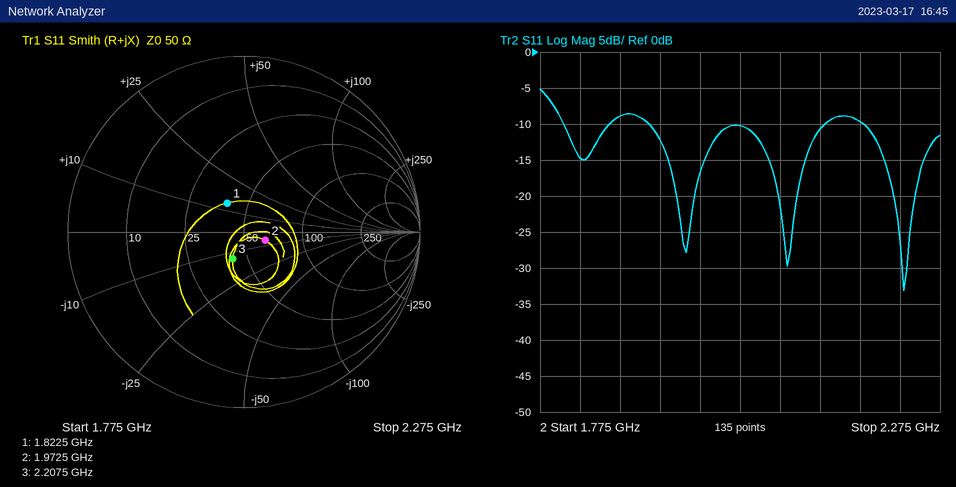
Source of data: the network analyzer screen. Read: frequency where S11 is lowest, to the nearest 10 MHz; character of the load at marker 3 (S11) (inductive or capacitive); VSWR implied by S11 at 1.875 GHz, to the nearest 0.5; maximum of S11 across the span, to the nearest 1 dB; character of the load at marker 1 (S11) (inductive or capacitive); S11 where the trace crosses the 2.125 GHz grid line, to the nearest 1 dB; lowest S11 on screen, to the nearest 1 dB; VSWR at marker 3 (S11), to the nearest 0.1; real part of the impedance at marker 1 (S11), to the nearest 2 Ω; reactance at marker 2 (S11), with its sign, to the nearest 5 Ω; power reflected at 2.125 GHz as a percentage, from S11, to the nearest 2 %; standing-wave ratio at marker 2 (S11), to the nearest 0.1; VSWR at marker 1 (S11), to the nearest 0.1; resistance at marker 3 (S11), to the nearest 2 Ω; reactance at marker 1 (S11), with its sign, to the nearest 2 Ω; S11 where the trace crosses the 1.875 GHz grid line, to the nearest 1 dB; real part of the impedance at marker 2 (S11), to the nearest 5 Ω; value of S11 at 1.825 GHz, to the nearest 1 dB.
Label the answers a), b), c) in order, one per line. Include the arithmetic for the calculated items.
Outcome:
a) 2.23 GHz
b) capacitive
c) |Γ| = 10^(-9/20) = 0.3548; VSWR = (1 + 0.3548)/(1 − 0.3548) ≈ 2.10, so 2.0 to the nearest 0.5
d) -5 dB
e) inductive
f) -11 dB
g) -33 dB
h) 1.4
i) 40 Ω
j) -5 Ω
k) 10^(-11/10) ≈ 8 %
l) 1.3
m) 1.5
n) 42 Ω
o) +14 Ω
p) -9 dB
q) 65 Ω
r) -15 dB
